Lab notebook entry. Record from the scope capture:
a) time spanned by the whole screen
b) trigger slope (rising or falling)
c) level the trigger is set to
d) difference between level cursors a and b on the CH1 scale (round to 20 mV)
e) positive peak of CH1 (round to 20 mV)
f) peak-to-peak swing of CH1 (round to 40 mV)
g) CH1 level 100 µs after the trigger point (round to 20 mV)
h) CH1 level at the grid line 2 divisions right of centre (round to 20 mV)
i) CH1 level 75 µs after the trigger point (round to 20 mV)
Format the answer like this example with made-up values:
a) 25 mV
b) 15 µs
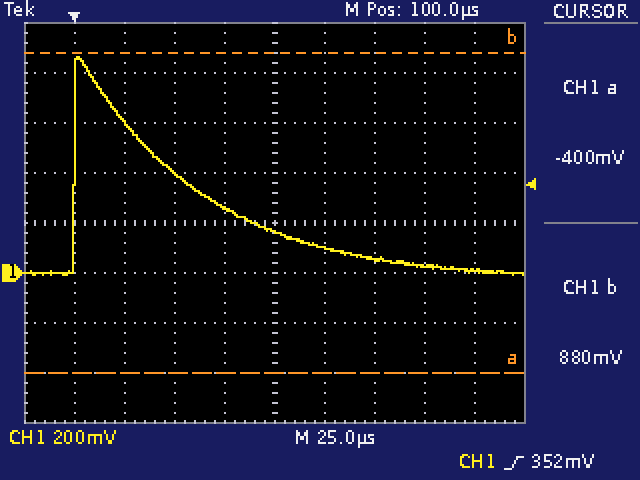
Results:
a) 250 µs
b) rising
c) 352 mV
d) 1.28 V
e) 860 mV
f) 880 mV
g) 160 mV
h) 60 mV
i) 260 mV
